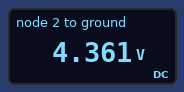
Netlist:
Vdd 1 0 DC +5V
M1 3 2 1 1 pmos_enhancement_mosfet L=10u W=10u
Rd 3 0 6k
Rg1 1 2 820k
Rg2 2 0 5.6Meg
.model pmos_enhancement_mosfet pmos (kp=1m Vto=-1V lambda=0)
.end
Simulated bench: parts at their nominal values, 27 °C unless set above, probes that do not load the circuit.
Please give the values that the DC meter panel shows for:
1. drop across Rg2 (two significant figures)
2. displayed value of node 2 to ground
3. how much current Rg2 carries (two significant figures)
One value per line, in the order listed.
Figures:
4.4 V
4.361 V
780 nA
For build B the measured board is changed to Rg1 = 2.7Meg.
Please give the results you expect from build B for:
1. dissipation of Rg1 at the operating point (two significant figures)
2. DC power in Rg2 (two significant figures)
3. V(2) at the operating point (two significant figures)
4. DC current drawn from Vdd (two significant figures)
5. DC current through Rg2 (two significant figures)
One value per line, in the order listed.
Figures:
980 nW
2.0 µW
3.4 V
200 µA
600 nA
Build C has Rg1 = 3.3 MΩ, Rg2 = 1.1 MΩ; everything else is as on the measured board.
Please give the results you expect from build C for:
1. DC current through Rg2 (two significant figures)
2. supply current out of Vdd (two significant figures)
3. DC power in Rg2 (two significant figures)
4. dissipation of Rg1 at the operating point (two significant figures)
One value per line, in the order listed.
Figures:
1.1 µA
780 µA
1.4 µW
4.3 µW
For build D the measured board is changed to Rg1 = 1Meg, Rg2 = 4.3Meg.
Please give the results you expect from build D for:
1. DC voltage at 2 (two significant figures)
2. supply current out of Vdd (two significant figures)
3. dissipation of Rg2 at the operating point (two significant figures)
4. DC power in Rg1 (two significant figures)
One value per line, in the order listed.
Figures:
4.1 V
940 nA
3.8 µW
890 nW
